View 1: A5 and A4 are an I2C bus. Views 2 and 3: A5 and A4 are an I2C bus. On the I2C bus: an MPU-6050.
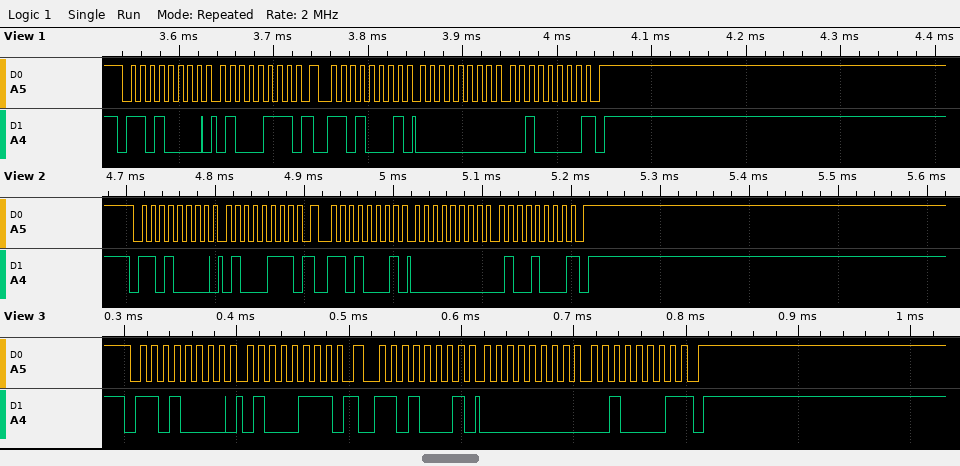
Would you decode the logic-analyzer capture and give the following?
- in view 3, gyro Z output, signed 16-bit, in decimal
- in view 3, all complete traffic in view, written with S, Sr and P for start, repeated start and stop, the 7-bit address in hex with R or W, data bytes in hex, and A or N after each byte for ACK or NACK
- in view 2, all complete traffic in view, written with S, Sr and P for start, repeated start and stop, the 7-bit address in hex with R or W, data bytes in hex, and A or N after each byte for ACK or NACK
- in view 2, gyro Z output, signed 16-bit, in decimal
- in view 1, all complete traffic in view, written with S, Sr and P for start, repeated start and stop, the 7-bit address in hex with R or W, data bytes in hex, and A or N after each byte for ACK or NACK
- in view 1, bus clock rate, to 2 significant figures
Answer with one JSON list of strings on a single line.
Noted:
["33", "S 68W A 47 A Sr 68R A 00 A 21 N P", "S 68W A 47 A Sr 68R A 00 A 48 N P", "72", "S 68W A 47 A Sr 68R A 00 A 20 N P", "100 kHz"]
